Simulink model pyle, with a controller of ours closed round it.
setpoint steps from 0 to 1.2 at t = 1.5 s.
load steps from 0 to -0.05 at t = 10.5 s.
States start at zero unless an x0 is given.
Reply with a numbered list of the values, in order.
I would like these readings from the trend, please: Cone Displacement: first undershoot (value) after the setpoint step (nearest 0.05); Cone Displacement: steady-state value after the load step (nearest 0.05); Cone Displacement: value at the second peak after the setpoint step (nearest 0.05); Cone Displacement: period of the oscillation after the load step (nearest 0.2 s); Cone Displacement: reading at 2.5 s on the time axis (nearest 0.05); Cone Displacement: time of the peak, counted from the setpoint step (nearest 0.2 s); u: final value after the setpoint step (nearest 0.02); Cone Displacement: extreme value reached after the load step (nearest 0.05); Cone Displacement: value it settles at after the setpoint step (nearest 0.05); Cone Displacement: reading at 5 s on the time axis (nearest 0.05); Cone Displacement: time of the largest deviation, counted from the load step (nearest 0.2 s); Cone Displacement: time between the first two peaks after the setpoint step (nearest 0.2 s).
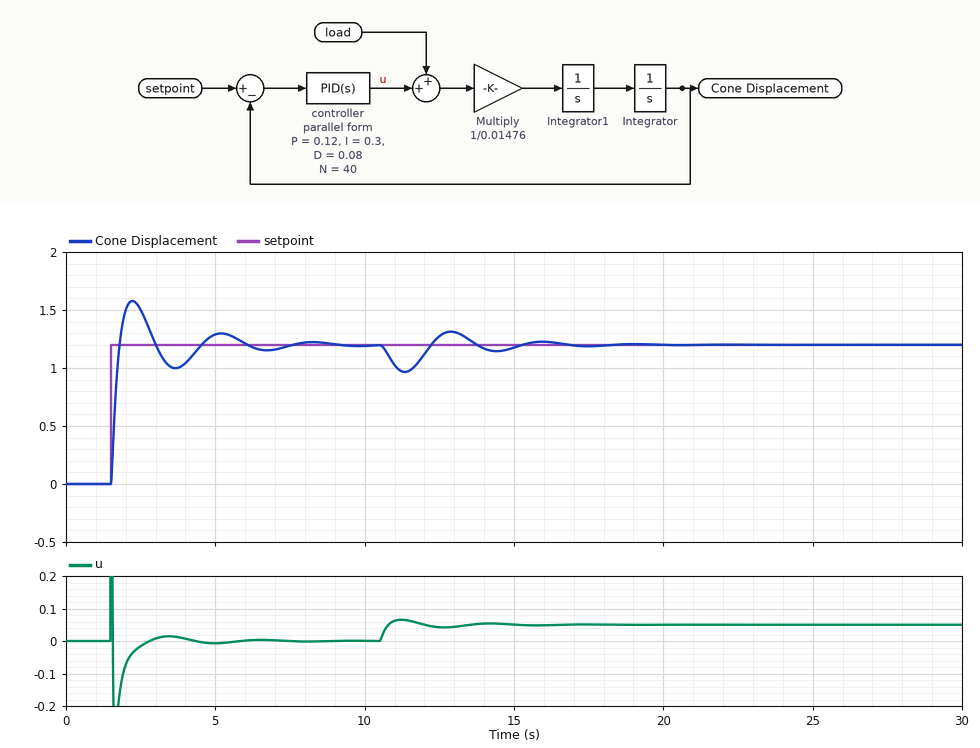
1. 1.00
2. 1.20
3. 1.30
4. 3.0 s
5. 1.50
6. 0.8 s
7. 0.00
8. 0.95
9. 1.20
10. 1.30
11. 0.8 s
12. 3.0 s
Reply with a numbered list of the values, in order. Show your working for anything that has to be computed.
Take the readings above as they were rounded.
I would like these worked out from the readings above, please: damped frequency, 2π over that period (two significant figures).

1. 2π / 3 = 2.1 rad/s
